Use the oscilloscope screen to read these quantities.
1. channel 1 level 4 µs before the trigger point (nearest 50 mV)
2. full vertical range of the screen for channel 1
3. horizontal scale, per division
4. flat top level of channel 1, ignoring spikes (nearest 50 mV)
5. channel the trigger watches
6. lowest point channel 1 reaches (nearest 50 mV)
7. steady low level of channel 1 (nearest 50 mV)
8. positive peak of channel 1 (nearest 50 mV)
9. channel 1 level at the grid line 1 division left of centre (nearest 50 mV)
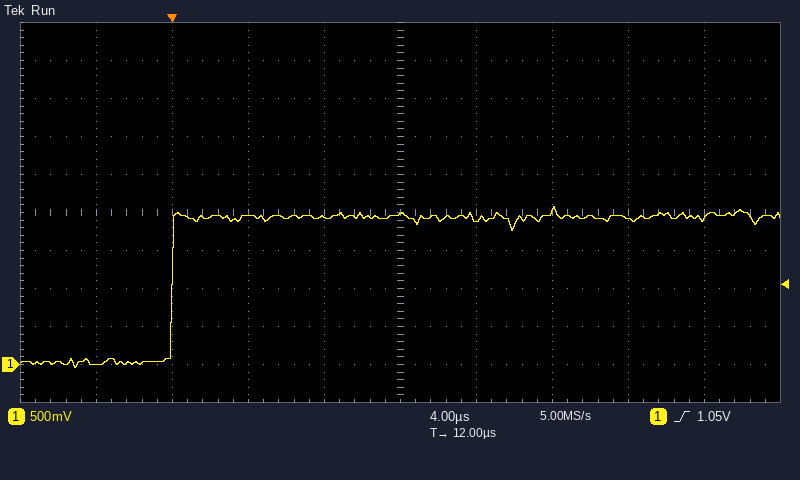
0 mV
5 V
4 µs
1.95 V
channel 1
-50 mV
50 mV
2.10 V
1.95 V
